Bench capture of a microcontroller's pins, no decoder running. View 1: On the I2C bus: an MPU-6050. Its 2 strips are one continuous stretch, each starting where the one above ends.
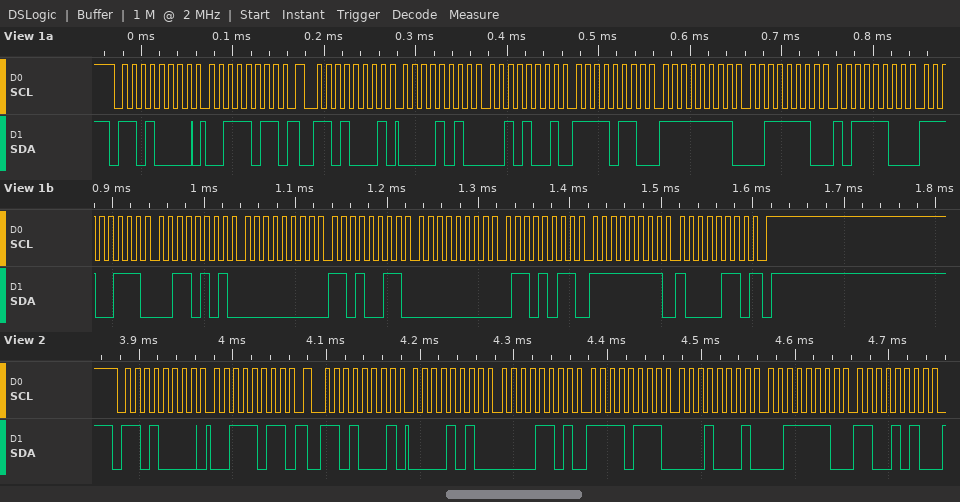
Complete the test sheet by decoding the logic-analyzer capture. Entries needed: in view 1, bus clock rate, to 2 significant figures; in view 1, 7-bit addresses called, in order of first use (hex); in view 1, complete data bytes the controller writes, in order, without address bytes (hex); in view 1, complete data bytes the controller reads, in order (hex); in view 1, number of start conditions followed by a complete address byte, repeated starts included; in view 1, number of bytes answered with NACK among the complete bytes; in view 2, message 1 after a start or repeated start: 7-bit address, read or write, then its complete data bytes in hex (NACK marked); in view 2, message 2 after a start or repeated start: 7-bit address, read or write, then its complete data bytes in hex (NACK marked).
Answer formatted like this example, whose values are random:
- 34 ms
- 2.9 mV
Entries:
- 100 kHz
- 0x68
- 3B
- 0A 29 F6 FF 3E BC E7 35 00 D3 00 6B FF 86
- 2
- 1
- 0x68 write: 3B
- 0x68 read: 0A 0D F7 11 3E CA
